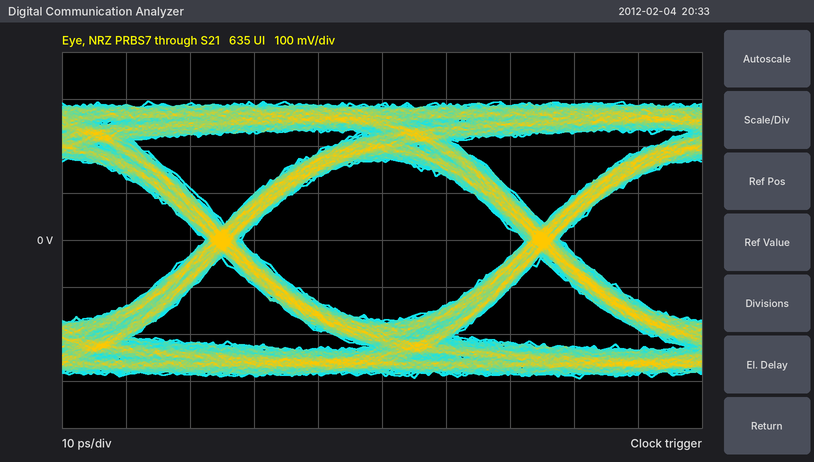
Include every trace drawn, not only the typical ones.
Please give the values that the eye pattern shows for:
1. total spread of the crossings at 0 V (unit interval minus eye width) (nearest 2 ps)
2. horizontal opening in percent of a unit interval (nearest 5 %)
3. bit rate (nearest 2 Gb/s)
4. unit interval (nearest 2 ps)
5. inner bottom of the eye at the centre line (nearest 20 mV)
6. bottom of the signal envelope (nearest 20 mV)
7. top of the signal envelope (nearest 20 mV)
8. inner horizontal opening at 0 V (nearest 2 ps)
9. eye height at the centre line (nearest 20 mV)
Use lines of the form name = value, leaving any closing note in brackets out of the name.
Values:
total spread of the crossings at 0 V (unit interval minus eye width) = 6 ps
horizontal opening in percent of a unit interval = 90 %
bit rate = 20 Gb/s
unit interval = 50 ps
inner bottom of the eye at the centre line = -180 mV
bottom of the signal envelope = -300 mV
top of the signal envelope = 300 mV
inner horizontal opening at 0 V = 44 ps
eye height at the centre line = 340 mV
